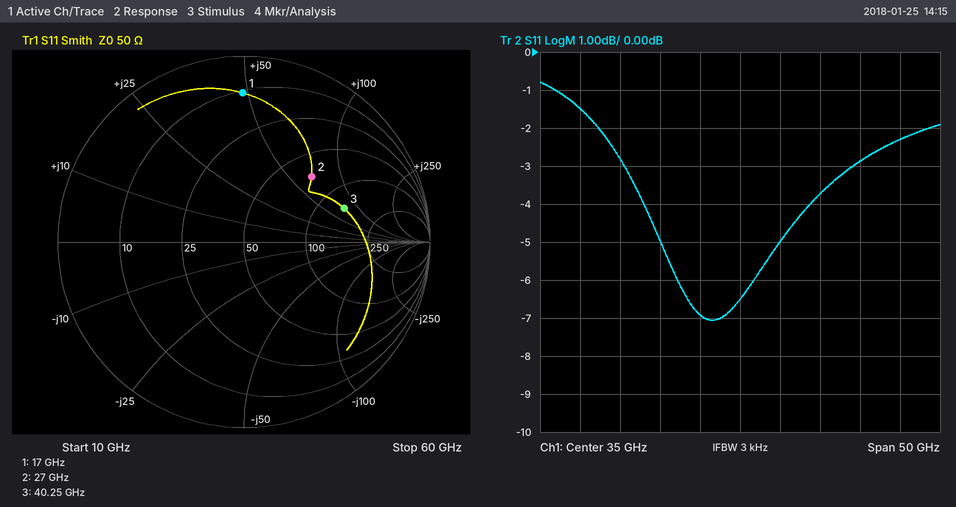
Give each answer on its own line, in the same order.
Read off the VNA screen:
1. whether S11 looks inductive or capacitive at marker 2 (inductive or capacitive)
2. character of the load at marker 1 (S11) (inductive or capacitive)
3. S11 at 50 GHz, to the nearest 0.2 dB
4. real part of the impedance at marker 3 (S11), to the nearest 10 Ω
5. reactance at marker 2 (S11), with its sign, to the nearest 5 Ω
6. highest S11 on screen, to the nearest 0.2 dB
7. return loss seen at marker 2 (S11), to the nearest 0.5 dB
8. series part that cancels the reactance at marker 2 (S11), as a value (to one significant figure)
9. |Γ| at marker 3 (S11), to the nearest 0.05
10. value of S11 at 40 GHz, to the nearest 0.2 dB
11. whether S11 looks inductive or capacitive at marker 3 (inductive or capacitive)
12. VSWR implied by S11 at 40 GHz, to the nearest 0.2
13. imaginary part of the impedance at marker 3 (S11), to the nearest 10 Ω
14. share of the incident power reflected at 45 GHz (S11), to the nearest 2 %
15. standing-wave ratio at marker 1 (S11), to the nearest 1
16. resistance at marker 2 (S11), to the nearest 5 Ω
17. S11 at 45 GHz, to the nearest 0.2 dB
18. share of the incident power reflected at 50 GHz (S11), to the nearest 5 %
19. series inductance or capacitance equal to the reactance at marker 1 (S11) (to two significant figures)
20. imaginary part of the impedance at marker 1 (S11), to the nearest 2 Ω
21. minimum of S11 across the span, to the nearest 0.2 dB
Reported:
inductive
inductive
-2.8 dB
140 Ω
+65 Ω
-0.8 dB
6.0 dB
90 fF
0.55
-5.0 dB
inductive
3.6
+70 Ω
42 %
9
70 Ω
-3.8 dB
50 %
450 pH
+48 Ω
-7.0 dB
